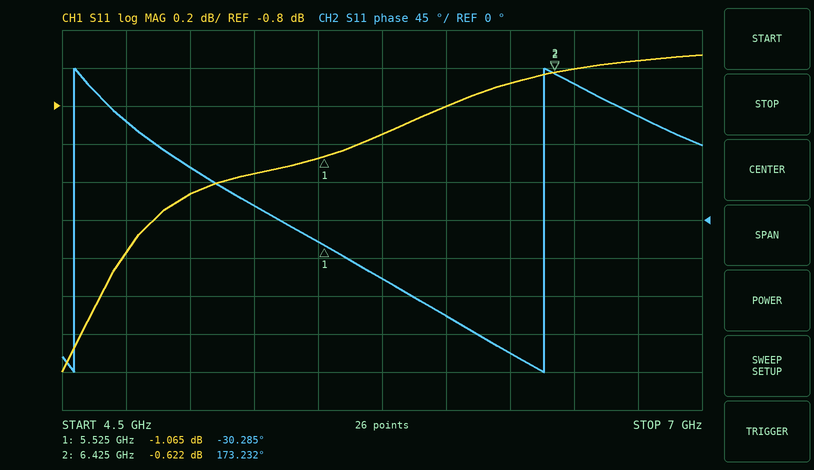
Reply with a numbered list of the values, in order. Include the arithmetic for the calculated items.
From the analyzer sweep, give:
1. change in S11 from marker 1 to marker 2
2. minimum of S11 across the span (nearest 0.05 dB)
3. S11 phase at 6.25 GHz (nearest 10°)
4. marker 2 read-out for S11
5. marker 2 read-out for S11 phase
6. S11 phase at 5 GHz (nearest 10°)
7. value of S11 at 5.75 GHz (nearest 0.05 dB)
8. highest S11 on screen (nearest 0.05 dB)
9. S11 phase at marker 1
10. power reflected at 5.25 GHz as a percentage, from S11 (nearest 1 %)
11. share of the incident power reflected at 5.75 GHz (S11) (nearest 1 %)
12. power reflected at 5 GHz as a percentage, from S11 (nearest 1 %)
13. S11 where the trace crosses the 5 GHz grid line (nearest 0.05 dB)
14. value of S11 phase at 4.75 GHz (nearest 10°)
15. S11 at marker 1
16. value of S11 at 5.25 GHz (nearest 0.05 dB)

1. -0.622 − (-1.065) = 0.443 dB
2. -2.20 dB
3. -160°
4. -0.622 dB
5. 173.232°
6. 60°
7. -0.95 dB
8. -0.55 dB
9. -30.285°
10. 10^(-1.15/10) ≈ 77 %
11. 10^(-0.95/10) ≈ 80 %
12. 10^(-1.25/10) ≈ 75 %
13. -1.25 dB
14. 120°
15. -1.065 dB
16. -1.15 dB
